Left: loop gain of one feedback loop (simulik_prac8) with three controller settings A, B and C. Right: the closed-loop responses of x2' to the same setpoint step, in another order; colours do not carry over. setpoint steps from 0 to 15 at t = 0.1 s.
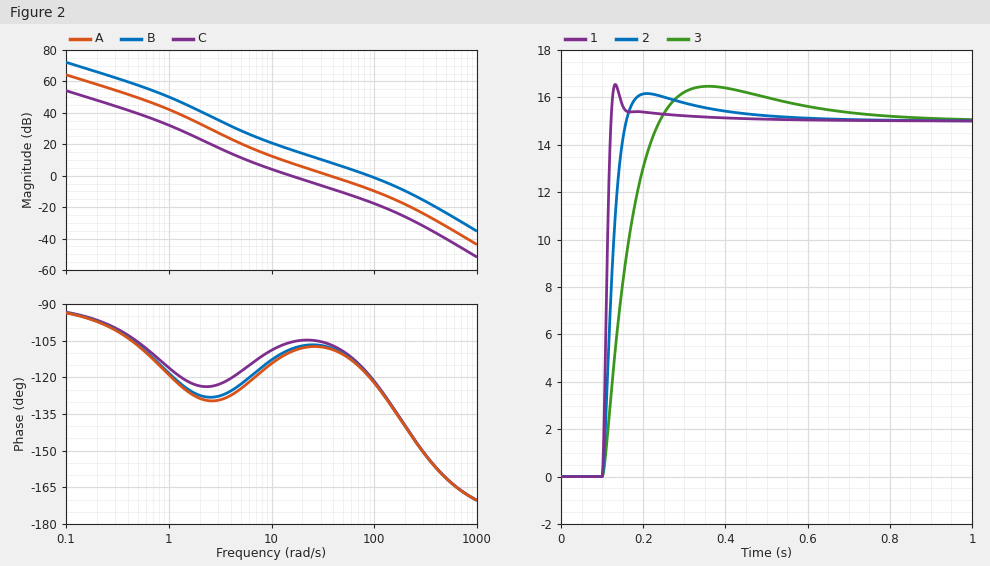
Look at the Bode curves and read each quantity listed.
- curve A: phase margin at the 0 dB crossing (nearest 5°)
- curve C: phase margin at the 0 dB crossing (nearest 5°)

70°
75°
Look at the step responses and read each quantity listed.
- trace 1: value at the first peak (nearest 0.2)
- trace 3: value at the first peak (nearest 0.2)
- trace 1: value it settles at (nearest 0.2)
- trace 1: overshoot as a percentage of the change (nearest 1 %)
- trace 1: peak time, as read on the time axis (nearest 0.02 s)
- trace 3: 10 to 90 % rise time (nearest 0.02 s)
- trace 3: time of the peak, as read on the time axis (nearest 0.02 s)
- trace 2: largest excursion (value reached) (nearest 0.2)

16.6
16.4
15.0
10 %
0.14 s
0.10 s
0.36 s
16.2
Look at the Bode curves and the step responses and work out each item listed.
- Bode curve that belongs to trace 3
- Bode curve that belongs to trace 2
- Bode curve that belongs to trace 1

C
A
B
